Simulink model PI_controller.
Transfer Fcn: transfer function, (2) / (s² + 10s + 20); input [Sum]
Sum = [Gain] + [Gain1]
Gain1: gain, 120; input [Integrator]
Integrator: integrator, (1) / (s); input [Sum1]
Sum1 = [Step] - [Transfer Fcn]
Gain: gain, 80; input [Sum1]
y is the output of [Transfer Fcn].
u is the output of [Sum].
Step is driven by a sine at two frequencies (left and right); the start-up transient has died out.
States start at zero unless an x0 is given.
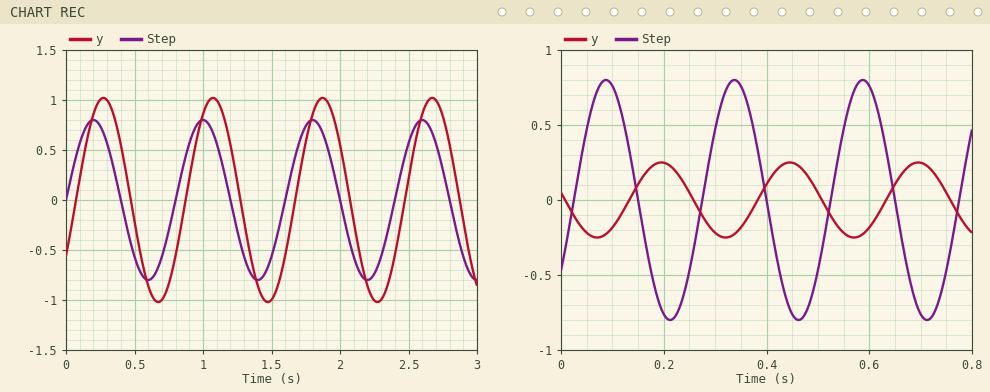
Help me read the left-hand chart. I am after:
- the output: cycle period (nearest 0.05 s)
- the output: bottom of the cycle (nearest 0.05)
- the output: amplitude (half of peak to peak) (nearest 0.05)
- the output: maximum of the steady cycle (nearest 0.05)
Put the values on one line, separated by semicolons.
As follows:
0.80 s; -1.00; 1.00; 1.00
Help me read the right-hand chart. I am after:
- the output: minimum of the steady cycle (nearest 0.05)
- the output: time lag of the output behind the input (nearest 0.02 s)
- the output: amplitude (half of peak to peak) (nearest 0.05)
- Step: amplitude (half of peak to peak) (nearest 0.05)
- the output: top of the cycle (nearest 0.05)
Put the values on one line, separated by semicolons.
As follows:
-0.25; 0.10 s; 0.25; 0.80; 0.25
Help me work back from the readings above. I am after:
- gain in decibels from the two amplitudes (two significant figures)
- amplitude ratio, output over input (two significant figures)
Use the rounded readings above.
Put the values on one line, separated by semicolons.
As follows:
-10 dB; 0.31
